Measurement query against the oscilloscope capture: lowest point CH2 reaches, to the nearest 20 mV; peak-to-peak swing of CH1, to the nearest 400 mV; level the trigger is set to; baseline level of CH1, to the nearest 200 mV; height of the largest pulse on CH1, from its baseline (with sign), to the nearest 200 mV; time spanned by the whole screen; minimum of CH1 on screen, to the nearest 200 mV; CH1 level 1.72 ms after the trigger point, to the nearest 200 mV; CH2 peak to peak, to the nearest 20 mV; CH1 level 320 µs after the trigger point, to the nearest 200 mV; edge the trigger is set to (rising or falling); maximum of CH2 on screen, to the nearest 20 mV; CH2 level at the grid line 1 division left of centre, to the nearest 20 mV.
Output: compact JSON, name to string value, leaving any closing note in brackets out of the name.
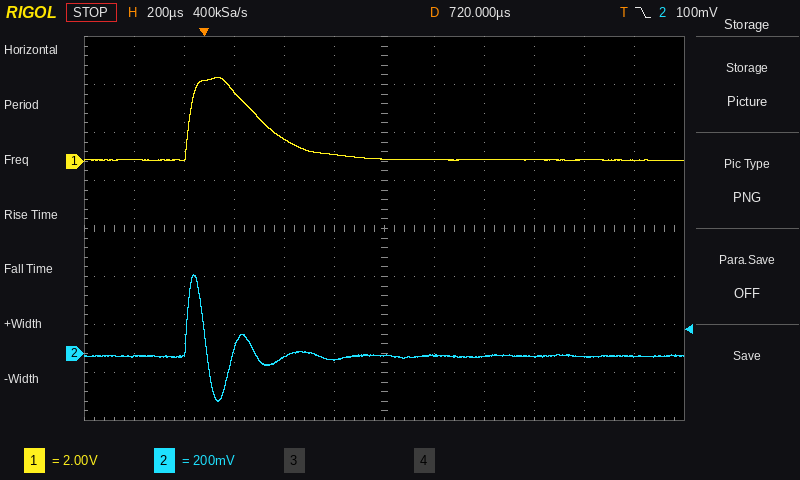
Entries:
{"lowest point CH2 reaches, to the nearest 20 mV": "-200 mV", "peak-to-peak swing of CH1, to the nearest 400 mV": "3.6 V", "level the trigger is set to": "100 mV", "baseline level of CH1, to the nearest 200 mV": "0.0 V", "height of the largest pulse on CH1, from its baseline (with sign), to the nearest 200 mV": "+3.4 V", "time spanned by the whole screen": "2.4 ms", "minimum of CH1 on screen, to the nearest 200 mV": "0.0 V", "CH1 level 1.72 ms after the trigger point, to the nearest 200 mV": "0.0 V", "CH2 peak to peak, to the nearest 20 mV": "520 mV", "CH1 level 320 µs after the trigger point, to the nearest 200 mV": "1.0 V", "edge the trigger is set to": "falling", "maximum of CH2 on screen, to the nearest 20 mV": "320 mV", "CH2 level at the grid line 1 division left of centre, to the nearest 20 mV": "-20 mV"}
